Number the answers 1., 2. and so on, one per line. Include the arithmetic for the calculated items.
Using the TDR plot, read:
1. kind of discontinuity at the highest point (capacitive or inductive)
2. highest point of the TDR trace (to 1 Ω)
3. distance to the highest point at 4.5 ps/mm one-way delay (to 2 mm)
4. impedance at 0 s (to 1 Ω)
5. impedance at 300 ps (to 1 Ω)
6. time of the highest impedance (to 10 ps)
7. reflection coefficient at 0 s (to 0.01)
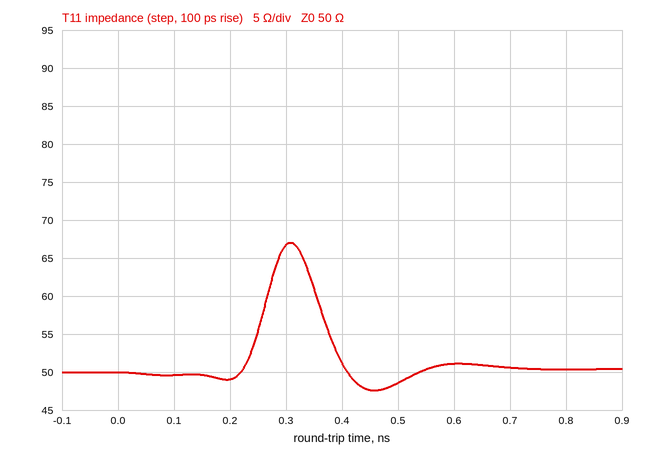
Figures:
1. inductive
2. 67 Ω
3. 310 ps / 2 / 4.5 ps/mm ≈ 34 mm
4. 50 Ω
5. 67 Ω
6. 310 ps
7. (50 − 50)/(50 + 50) ≈ 0.00
